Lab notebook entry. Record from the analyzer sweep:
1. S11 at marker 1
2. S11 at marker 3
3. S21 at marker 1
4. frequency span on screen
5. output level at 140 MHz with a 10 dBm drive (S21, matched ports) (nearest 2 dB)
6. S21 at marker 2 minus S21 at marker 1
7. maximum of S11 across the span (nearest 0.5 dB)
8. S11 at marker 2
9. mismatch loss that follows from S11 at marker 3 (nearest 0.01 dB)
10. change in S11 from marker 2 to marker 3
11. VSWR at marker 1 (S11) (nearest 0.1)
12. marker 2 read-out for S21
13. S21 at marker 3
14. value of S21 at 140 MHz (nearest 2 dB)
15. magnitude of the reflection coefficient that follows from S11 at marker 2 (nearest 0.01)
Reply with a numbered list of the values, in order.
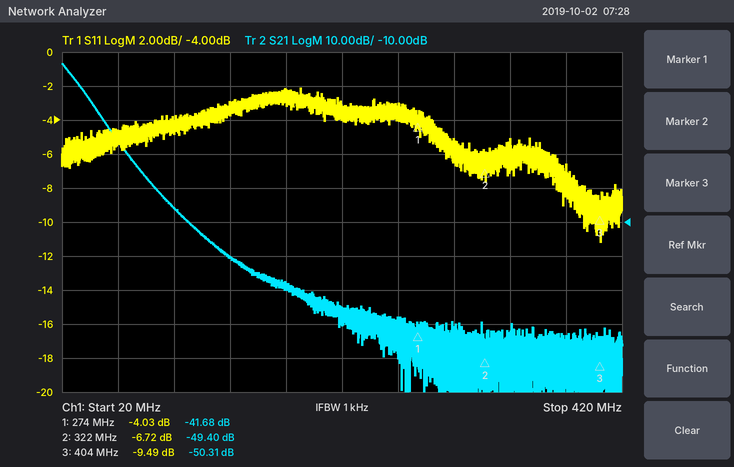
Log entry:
1. -4.03 dB
2. -9.49 dB
3. -41.68 dB
4. 400 MHz
5. -10 dBm
6. -7.72 dB
7. -2.0 dB
8. -6.72 dB
9. 0.52 dB
10. -2.77 dB
11. 4.4
12. -49.40 dB
13. -50.31 dB
14. -20 dB
15. 0.46
